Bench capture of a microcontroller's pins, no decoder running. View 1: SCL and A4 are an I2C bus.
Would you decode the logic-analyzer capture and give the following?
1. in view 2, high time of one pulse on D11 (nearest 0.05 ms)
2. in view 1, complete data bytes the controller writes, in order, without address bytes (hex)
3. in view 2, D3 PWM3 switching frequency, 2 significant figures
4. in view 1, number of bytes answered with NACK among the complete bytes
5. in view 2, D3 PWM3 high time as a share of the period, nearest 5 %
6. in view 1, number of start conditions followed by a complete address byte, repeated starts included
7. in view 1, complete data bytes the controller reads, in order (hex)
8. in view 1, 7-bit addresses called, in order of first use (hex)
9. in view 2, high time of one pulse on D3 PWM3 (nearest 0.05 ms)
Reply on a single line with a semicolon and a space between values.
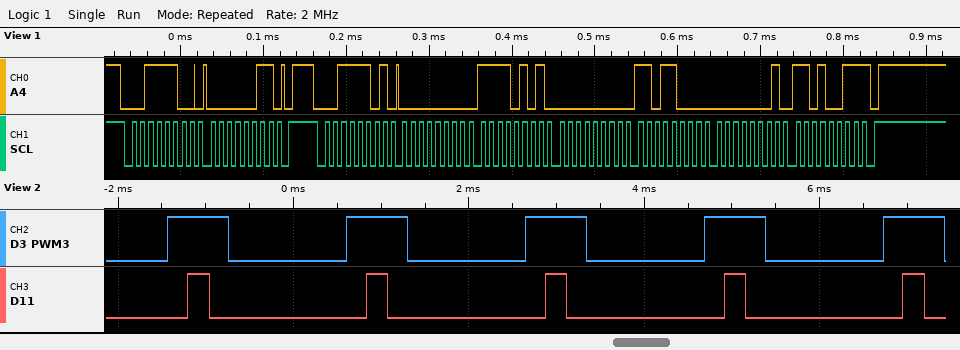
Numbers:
0.25 ms; 03; 490 Hz; 1; 35 %; 2; 00 F5 00 D8 01 D3; 0x1E; 0.70 ms
